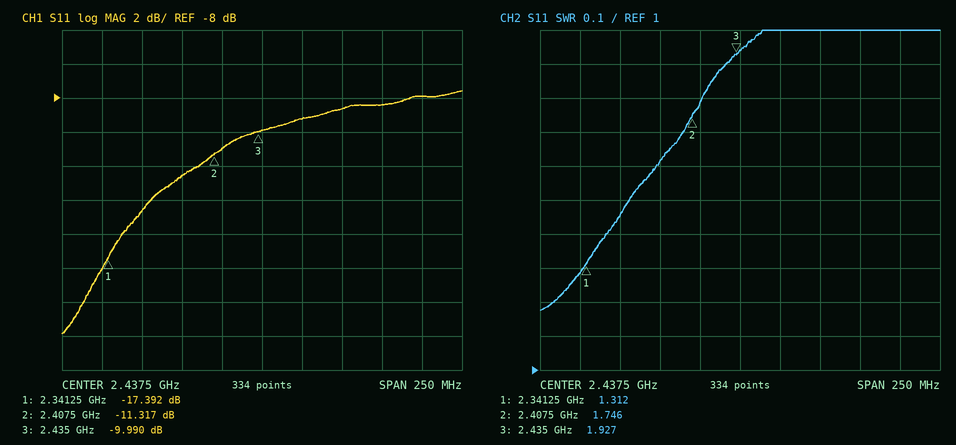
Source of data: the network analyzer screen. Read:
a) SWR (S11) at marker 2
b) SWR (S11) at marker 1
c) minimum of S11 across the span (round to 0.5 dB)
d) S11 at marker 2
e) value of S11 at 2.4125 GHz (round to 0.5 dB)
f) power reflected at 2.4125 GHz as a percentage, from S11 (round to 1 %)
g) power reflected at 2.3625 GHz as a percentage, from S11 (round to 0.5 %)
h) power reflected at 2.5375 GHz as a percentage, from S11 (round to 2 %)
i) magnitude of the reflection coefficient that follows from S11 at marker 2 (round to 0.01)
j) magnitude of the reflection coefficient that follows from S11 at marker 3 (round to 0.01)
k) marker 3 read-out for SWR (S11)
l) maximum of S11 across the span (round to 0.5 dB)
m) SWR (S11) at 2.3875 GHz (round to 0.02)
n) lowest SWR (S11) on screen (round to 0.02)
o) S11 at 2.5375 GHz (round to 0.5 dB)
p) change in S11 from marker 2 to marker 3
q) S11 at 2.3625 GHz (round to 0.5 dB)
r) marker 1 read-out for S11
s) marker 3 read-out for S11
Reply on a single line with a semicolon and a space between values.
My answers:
1.746; 1.312; -22.0 dB; -11.317 dB; -11.0 dB; 8 %; 3.5 %; 16 %; 0.27; 0.32; 1.927; -7.5 dB; 1.62; 1.18; -8.0 dB; 1.327 dB; -14.5 dB; -17.392 dB; -9.990 dB
